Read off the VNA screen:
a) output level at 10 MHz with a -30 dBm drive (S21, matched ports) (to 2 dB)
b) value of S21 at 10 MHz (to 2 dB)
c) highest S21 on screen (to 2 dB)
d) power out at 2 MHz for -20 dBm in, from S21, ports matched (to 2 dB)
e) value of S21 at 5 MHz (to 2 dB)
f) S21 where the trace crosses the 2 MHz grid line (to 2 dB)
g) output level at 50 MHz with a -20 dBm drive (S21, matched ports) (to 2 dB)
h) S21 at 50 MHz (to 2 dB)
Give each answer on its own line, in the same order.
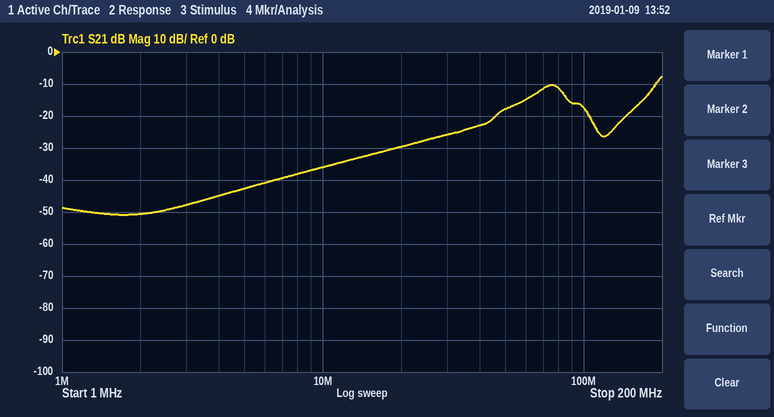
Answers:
-66 dBm
-36 dB
-8 dB
-70 dBm
-42 dB
-50 dB
-38 dBm
-18 dB
